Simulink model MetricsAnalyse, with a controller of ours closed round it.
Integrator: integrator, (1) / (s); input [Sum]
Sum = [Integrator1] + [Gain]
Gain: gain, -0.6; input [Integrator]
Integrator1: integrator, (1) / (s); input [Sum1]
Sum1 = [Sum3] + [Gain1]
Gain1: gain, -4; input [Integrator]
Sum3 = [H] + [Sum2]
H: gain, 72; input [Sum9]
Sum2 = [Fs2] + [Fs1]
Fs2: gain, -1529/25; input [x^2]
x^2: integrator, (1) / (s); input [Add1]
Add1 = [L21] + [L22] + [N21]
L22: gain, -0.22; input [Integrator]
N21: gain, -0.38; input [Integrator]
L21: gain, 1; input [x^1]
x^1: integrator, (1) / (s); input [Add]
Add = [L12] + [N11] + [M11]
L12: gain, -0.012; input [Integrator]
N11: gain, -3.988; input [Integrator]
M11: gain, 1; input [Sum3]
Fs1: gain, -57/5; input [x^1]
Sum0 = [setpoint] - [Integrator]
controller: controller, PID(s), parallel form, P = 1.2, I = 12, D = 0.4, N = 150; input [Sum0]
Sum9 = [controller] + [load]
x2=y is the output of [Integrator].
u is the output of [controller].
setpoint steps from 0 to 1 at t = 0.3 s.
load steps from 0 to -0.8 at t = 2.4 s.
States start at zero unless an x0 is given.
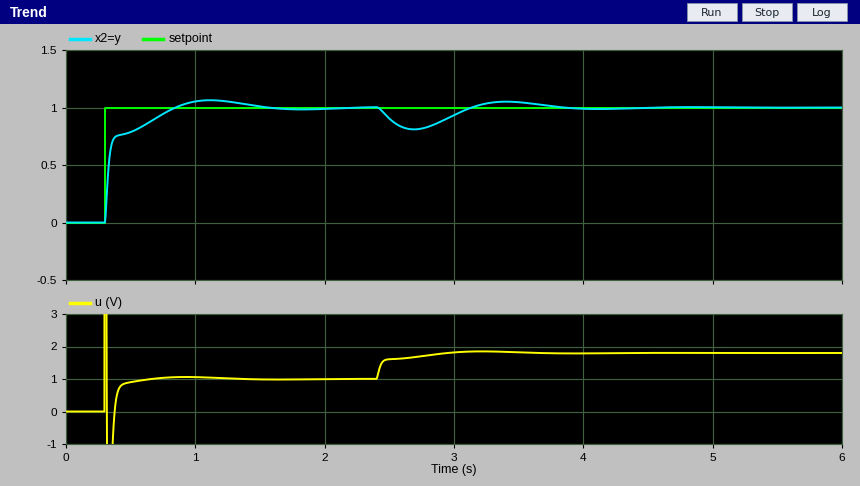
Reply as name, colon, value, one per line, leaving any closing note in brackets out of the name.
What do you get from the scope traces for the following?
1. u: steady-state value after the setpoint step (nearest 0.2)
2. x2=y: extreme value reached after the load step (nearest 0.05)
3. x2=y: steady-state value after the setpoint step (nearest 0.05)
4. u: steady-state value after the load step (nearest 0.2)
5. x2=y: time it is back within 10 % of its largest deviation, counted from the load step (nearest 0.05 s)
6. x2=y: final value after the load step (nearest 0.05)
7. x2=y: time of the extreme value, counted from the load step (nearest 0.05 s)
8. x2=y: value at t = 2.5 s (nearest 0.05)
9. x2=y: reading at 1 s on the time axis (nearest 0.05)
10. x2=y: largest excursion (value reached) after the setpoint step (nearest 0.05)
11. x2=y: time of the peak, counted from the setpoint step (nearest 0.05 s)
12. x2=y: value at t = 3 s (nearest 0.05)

u: steady-state value after the setpoint step: 1.0
x2=y: extreme value reached after the load step: 0.80
x2=y: steady-state value after the setpoint step: 1.00
u: steady-state value after the load step: 1.8
x2=y: time it is back within 10 % of its largest deviation, counted from the load step: 1.30 s
x2=y: final value after the load step: 1.00
x2=y: time of the extreme value, counted from the load step: 0.30 s
x2=y: value at t = 2.5 s: 0.90
x2=y: reading at 1 s on the time axis: 1.05
x2=y: largest excursion (value reached) after the setpoint step: 1.05
x2=y: time of the peak, counted from the setpoint step: 0.80 s
x2=y: value at t = 3 s: 0.95
